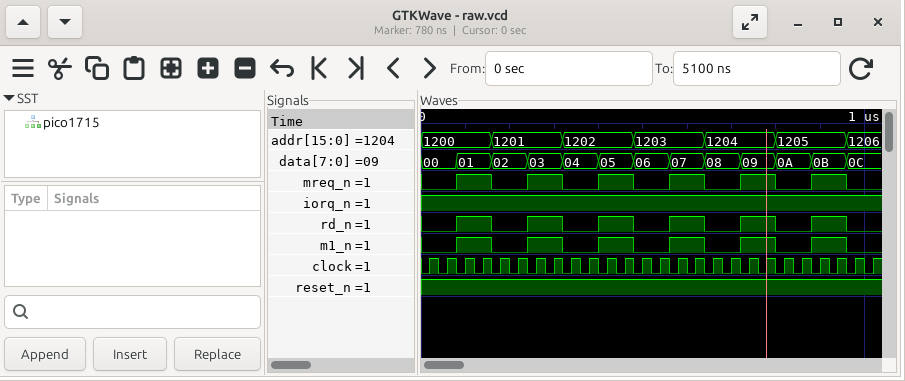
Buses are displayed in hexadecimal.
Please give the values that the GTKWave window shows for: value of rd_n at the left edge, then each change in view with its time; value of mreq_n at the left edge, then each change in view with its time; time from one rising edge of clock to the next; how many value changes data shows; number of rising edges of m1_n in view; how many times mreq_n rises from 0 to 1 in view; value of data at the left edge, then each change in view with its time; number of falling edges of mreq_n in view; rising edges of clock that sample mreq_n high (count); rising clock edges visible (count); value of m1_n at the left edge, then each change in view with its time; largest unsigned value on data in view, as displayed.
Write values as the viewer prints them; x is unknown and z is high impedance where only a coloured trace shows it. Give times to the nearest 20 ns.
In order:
0, 1 at 80 ns, 0 at 160 ns, 1 at 240 ns, 0 at 320 ns, 1 at 400 ns, 0 at 480 ns, 1 at 560 ns, 0 at 640 ns, 1 at 720 ns, 0 at 800 ns, 1 at 880 ns, 0 at 960 ns
0, 1 at 80 ns, 0 at 160 ns, 1 at 240 ns, 0 at 320 ns, 1 at 400 ns, 0 at 480 ns, 1 at 560 ns, 0 at 640 ns, 1 at 720 ns, 0 at 800 ns, 1 at 880 ns, 0 at 960 ns
40 ns
12
6
6
00, 01 at 80 ns, 02 at 160 ns, 03 at 240 ns, 04 at 320 ns, 05 at 400 ns, 06 at 480 ns, 07 at 560 ns, 08 at 640 ns, 09 at 720 ns, 0A at 800 ns, 0B at 880 ns, 0C at 960 ns
6
12
26
0, 1 at 80 ns, 0 at 160 ns, 1 at 240 ns, 0 at 320 ns, 1 at 400 ns, 0 at 480 ns, 1 at 560 ns, 0 at 640 ns, 1 at 720 ns, 0 at 800 ns, 1 at 880 ns, 0 at 960 ns
0C
